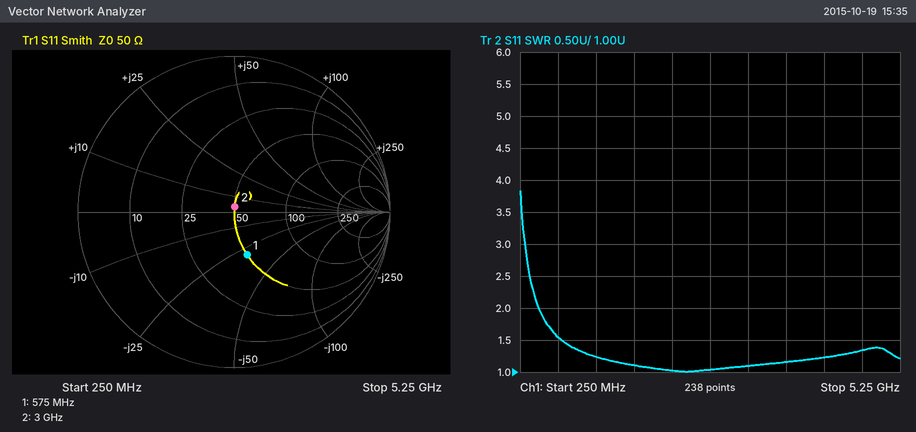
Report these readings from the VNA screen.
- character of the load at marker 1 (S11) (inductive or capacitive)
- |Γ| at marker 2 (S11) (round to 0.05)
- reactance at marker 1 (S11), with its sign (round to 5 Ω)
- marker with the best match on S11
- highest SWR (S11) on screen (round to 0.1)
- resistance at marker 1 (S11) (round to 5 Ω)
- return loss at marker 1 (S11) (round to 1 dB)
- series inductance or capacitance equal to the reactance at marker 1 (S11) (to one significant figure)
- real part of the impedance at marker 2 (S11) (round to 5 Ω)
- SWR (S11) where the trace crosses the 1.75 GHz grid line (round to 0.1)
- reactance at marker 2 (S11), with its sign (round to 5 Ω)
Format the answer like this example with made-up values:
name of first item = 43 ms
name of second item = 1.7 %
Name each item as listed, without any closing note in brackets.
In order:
character of the load at marker 1 (S11) = capacitive
|Γ| at marker 2 (S11) = 0.05
reactance at marker 1 (S11), with its sign = -30 Ω
marker with the best match on S11 = marker 2
highest SWR (S11) on screen = 3.8
resistance at marker 1 (S11) = 50 Ω
return loss at marker 1 (S11) = 11 dB
series inductance or capacitance equal to the reactance at marker 1 (S11) = 9 pF
real part of the impedance at marker 2 (S11) = 50 Ω
SWR (S11) where the trace crosses the 1.75 GHz grid line = 1.1
reactance at marker 2 (S11), with its sign = +5 Ω
